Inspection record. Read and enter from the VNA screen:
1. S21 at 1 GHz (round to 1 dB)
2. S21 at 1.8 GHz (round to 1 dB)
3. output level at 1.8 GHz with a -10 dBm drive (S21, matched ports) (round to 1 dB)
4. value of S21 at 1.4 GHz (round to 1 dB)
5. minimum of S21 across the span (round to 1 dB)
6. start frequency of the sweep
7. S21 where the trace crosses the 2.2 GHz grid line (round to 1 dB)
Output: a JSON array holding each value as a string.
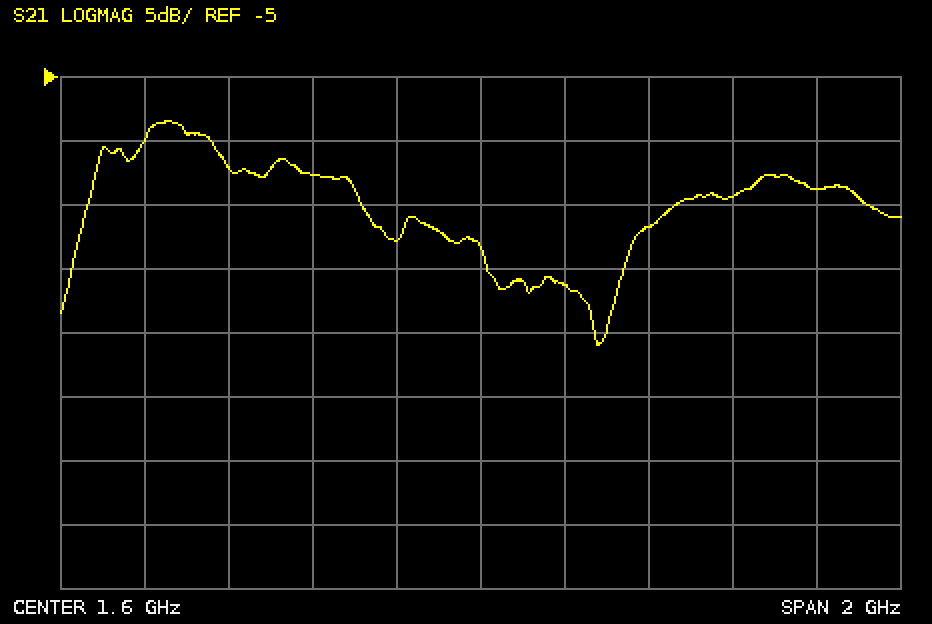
["-12 dB", "-21 dB", "-31 dBm", "-18 dB", "-26 dB", "600 MHz", "-14 dB"]
